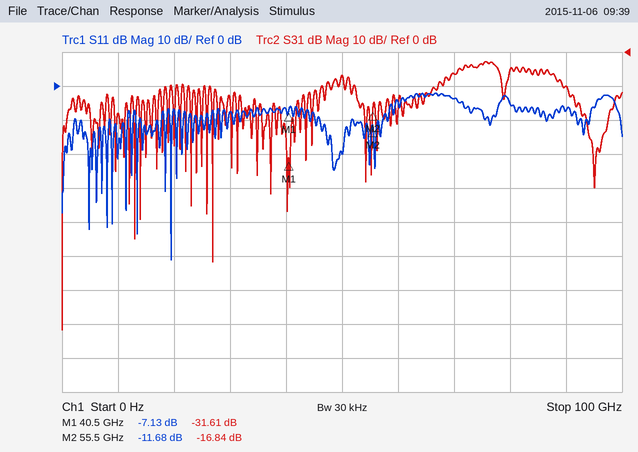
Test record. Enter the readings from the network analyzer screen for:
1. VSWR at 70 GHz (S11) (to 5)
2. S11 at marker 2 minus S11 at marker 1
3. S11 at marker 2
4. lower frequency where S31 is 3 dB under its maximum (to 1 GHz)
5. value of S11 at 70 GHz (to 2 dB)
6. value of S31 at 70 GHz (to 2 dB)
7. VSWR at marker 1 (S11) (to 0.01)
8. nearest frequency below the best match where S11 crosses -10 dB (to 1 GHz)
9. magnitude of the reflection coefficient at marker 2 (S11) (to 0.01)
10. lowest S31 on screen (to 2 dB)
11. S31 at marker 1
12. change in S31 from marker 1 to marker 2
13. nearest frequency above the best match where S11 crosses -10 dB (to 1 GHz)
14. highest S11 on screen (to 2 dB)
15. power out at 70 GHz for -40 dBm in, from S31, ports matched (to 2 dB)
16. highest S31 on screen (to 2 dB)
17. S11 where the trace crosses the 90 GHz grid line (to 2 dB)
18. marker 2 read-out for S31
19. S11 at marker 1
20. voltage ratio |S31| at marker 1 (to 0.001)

5
-4.55 dB
-11.68 dB
71 GHz
-4 dB
-6 dB
2.57
19 GHz
0.26
-82 dB
-31.61 dB
14.77 dB
20 GHz
-2 dB
-46 dBm
-2 dB
-8 dB
-16.84 dB
-7.13 dB
0.026
